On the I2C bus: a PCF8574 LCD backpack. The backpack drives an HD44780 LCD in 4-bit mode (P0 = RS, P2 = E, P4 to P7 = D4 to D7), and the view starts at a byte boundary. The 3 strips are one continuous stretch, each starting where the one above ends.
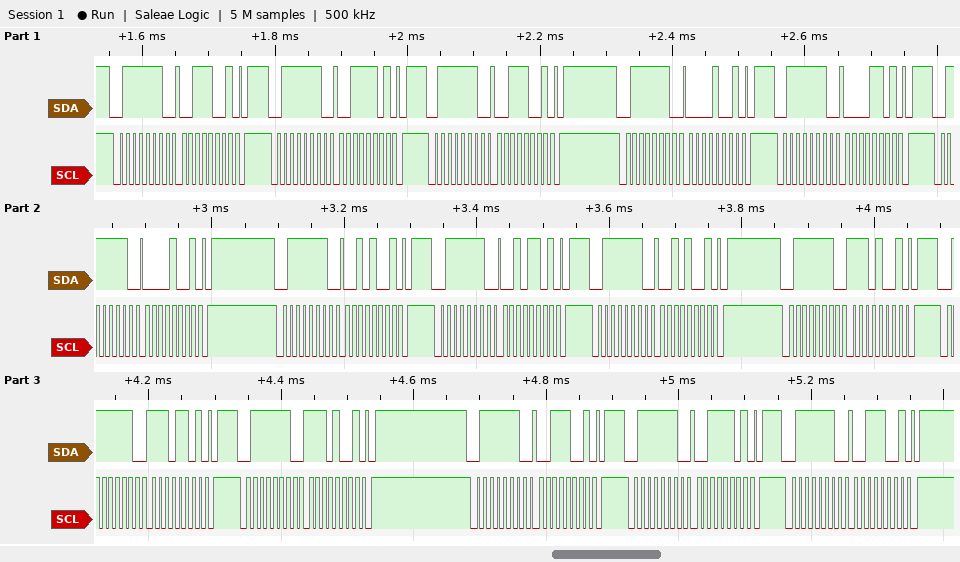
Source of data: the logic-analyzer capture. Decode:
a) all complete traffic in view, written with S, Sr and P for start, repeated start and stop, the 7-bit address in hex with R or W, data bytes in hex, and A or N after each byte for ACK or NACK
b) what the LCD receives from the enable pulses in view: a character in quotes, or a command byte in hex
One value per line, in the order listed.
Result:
S 3FW A 39 A P S 3FW A 3D A P S 3FW A 39 A P S 3FW A 09 A P S 3FW A 0D A P S 3FW A 09 A P S 3FW A 29 A P S 3FW A 2D A P S 3FW A 29 A P S 3FW A E9 A P S 3FW A ED A P S 3FW A E9 A P S 3FW A 39 A P S 3FW A 3D A P S 3FW A 39 A P
'0' '.'
